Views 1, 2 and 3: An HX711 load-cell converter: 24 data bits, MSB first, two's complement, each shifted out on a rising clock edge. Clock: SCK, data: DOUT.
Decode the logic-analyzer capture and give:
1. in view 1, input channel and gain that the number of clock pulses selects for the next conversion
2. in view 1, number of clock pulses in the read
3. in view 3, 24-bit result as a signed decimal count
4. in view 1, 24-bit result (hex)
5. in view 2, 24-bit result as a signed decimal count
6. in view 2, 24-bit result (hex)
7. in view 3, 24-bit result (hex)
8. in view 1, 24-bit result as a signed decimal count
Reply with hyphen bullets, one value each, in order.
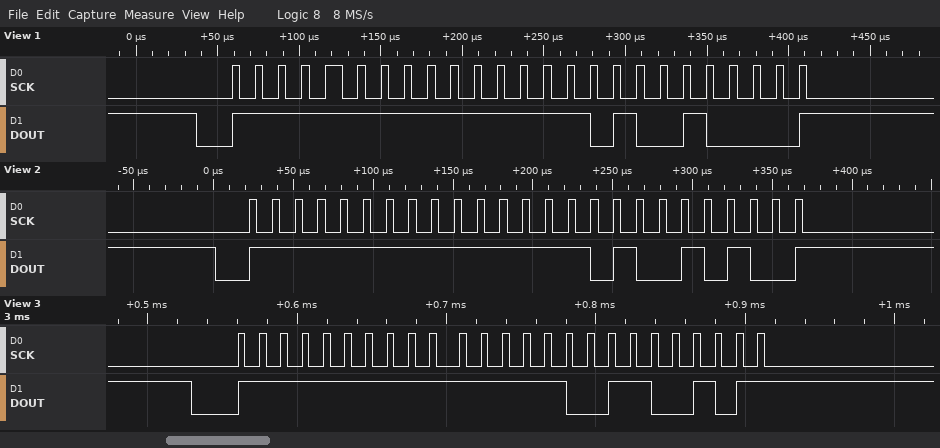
- channel A, gain 128
- 25
- -411
- 0xFFFE90
- -364
- 0xFFFE94
- 0xFFFE65
- -368
